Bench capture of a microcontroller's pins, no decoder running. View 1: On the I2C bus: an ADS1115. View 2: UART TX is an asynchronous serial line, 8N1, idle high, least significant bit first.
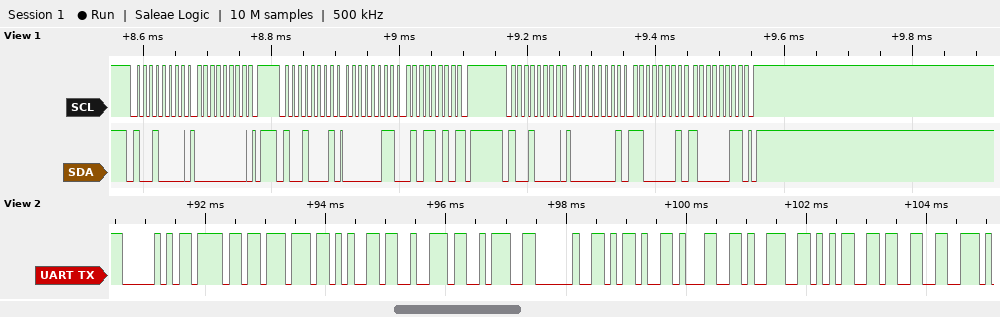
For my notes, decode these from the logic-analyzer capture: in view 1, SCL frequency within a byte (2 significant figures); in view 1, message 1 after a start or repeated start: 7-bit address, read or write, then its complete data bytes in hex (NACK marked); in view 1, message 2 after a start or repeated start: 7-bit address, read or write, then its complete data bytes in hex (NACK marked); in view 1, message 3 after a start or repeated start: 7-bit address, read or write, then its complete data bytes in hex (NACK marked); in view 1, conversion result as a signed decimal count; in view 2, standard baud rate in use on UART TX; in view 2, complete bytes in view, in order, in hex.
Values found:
100 kHz
0x48 write: 00
0x48 read: 03 5A NACK
0x48 write: 01 C1 83
858
9600 baud
50 6F 77 65 72 3A 20 2D 31 39 35 33
